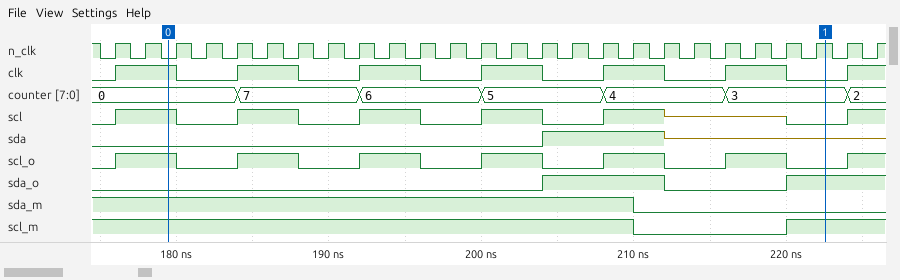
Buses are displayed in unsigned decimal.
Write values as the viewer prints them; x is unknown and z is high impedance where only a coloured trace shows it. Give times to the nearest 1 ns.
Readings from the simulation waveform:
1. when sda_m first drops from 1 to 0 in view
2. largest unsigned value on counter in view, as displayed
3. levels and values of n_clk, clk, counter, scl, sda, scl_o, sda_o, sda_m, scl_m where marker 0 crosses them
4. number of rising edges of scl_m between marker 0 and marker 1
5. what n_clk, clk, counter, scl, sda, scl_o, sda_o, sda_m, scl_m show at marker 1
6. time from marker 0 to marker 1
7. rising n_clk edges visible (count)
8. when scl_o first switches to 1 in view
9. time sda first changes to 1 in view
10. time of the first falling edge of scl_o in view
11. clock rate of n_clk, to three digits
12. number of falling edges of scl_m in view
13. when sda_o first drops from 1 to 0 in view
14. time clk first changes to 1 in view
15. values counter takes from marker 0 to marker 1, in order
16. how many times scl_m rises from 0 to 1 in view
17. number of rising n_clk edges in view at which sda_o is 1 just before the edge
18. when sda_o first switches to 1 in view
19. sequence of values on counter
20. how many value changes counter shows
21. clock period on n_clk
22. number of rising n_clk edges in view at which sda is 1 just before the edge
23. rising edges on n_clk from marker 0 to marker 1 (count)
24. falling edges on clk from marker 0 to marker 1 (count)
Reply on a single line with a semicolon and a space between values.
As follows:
210 ns; 7; n_clk=0, clk=1, counter=0, scl=1, sda=0, scl_o=1, sda_o=0, sda_m=1, scl_m=1; 1; n_clk=1, clk=0, counter=3, scl=0, sda=z, scl_o=0, sda_o=1, sda_m=0, scl_m=1; 43 ns; 26; 176 ns; 204 ns; 180 ns; 500 MHz; 1; 212 ns; 176 ns; 0, 7, 6, 5, 4, 3; 1; 7; 204 ns; 0, 7, 6, 5, 4, 3, 2; 6; 2 ns; 4; 22; 6
